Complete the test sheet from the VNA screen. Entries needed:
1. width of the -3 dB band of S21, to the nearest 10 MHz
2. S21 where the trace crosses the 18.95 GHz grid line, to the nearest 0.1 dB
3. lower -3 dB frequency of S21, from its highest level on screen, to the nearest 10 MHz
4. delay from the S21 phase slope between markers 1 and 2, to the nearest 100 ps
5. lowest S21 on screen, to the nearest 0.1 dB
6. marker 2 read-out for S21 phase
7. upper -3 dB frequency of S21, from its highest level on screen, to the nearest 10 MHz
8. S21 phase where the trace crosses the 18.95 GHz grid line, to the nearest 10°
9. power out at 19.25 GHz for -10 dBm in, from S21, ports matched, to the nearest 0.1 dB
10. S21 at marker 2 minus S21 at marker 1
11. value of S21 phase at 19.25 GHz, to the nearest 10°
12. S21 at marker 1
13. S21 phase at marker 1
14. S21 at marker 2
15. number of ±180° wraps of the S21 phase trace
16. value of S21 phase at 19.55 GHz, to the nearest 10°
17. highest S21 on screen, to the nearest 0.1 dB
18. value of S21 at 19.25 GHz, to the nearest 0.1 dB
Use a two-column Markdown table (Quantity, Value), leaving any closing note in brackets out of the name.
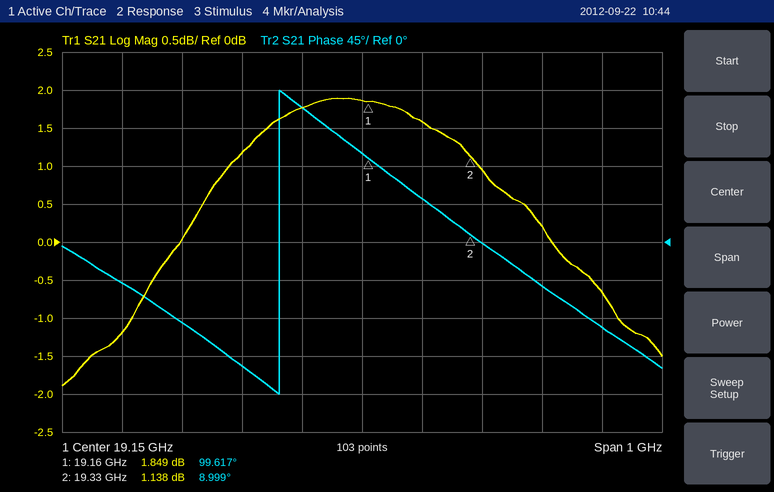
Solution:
| Quantity | Value |
|---|---|
| width of the -3 dB band of S21, to the nearest 10 MHz | 830 MHz |
| S21 where the trace crosses the 18.95 GHz grid line, to the nearest 0.1 dB | 1.2 dB |
| lower -3 dB frequency of S21, from its highest level on screen, to the nearest 10 MHz | 18.76 GHz |
| delay from the S21 phase slope between markers 1 and 2, to the nearest 100 ps | 1.5 ns |
| lowest S21 on screen, to the nearest 0.1 dB | -1.9 dB |
| marker 2 read-out for S21 phase | 8.999° |
| upper -3 dB frequency of S21, from its highest level on screen, to the nearest 10 MHz | 19.59 GHz |
| S21 phase where the trace crosses the 18.95 GHz grid line, to the nearest 10° | -150° |
| power out at 19.25 GHz for -10 dBm in, from S21, ports matched, to the nearest 0.1 dB | -8.4 dBm |
| S21 at marker 2 minus S21 at marker 1 | -0.711 dB |
| value of S21 phase at 19.25 GHz, to the nearest 10° | 50° |
| S21 at marker 1 | 1.849 dB |
| S21 phase at marker 1 | 99.617° |
| S21 at marker 2 | 1.138 dB |
| number of ±180° wraps of the S21 phase trace | 1 |
| value of S21 phase at 19.55 GHz, to the nearest 10° | -100° |
| highest S21 on screen, to the nearest 0.1 dB | 1.9 dB |
| value of S21 at 19.25 GHz, to the nearest 0.1 dB | 1.6 dB |
